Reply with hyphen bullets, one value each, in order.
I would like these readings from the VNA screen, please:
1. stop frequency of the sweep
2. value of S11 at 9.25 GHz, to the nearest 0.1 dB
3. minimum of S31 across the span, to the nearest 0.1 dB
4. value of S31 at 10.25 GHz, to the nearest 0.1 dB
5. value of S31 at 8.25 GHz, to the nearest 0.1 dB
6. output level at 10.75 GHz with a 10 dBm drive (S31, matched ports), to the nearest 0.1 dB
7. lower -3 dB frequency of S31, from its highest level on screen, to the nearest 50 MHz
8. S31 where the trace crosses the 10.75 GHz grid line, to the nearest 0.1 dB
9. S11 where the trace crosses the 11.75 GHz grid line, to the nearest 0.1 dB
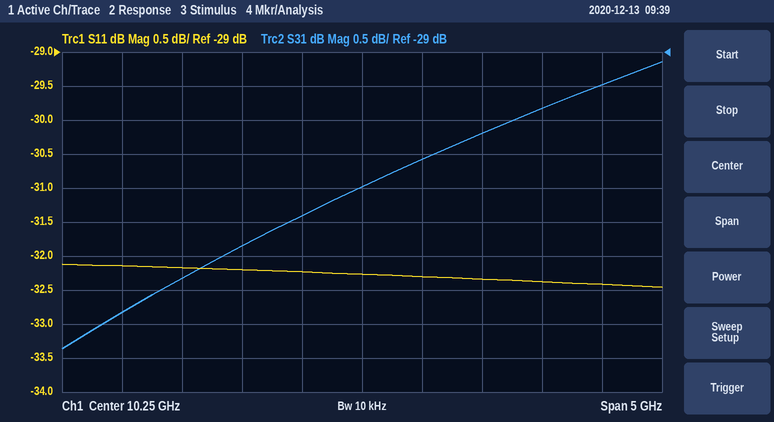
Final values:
- 12.75 GHz
- -32.2 dB
- -33.4 dB
- -31.0 dB
- -32.8 dB
- -20.6 dBm
- 8.95 GHz
- -30.6 dB
- -32.4 dB
